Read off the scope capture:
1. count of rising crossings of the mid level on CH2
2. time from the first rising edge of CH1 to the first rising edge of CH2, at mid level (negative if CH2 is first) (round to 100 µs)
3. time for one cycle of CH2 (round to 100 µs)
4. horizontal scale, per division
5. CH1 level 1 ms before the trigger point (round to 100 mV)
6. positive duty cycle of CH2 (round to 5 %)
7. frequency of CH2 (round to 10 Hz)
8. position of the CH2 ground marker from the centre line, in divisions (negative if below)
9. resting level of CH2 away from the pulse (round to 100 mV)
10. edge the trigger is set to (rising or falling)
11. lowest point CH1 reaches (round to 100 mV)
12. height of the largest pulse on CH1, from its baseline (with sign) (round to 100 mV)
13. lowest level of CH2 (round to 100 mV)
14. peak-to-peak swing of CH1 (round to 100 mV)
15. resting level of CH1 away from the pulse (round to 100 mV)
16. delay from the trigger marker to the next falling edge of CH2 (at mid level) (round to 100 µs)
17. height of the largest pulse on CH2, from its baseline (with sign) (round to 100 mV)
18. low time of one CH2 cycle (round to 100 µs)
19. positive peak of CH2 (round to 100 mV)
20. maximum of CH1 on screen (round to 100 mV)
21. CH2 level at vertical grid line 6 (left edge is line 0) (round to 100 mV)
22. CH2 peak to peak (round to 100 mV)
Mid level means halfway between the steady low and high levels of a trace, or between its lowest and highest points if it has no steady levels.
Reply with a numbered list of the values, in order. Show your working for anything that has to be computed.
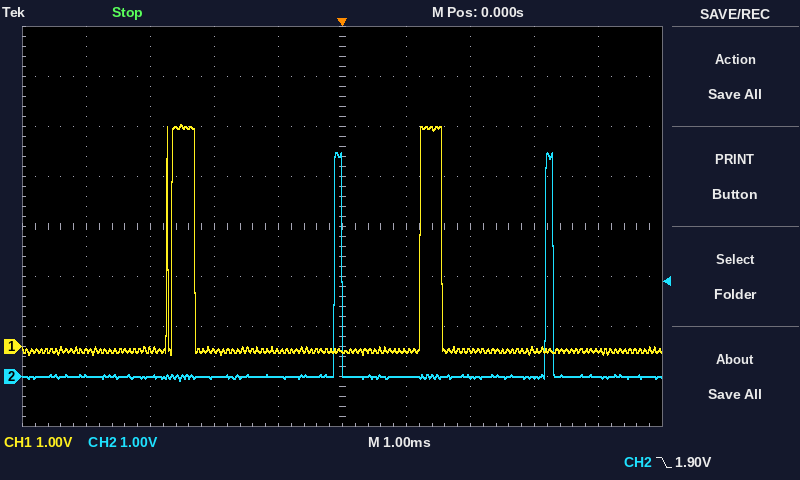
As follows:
1. 2
2. +2.5 ms
3. 3.3 ms
4. 1 ms
5. -100 mV
6. 5 %
7. 1 / 3.3 ms ≈ 303 Hz, so 300 Hz to the nearest 10 Hz
8. -3.0 div
9. 0.0 V
10. falling
11. -200 mV
12. 4.4 V − (-100 mV) = +4.5 V
13. -100 mV
14. 4.4 V − (-200 mV) = 4.6 V
15. -100 mV
16. 3.3 ms
17. 4.5 V − (0.0 V) = +4.5 V
18. 3.2 ms
19. 4.5 V
20. 4.4 V
21. 0.0 V
22. 4.5 V − (-100 mV) = 4.6 V
